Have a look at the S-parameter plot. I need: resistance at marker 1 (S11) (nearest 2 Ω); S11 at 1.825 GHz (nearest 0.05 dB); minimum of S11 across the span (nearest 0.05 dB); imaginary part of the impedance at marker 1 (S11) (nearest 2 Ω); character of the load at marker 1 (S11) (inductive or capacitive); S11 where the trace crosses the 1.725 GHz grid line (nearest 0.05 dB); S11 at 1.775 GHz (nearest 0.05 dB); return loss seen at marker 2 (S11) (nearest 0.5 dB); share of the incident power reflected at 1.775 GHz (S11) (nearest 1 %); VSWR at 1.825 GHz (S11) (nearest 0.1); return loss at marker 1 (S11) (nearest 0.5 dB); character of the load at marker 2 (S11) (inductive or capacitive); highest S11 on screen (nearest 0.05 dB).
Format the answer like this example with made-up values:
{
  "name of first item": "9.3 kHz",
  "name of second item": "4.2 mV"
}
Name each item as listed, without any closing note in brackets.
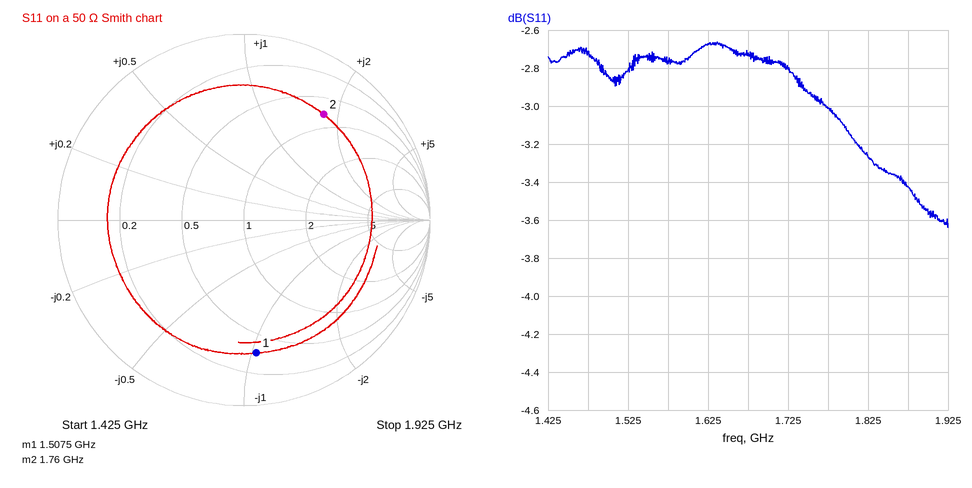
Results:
{
  "resistance at marker 1 (S11)": "18 Ω",
  "S11 at 1.825 GHz": "-3.25 dB",
  "minimum of S11 across the span": "-3.65 dB",
  "imaginary part of the impedance at marker 1 (S11)": "-52 Ω",
  "character of the load at marker 1 (S11)": "capacitive",
  "S11 where the trace crosses the 1.725 GHz grid line": "-2.80 dB",
  "S11 at 1.775 GHz": "-3.00 dB",
  "return loss seen at marker 2 (S11)": "3.0 dB",
  "share of the incident power reflected at 1.775 GHz (S11)": "50 %",
  "VSWR at 1.825 GHz (S11)": "5.4",
  "return loss at marker 1 (S11)": "3.0 dB",
  "character of the load at marker 2 (S11)": "inductive",
  "highest S11 on screen": "-2.65 dB"
}
